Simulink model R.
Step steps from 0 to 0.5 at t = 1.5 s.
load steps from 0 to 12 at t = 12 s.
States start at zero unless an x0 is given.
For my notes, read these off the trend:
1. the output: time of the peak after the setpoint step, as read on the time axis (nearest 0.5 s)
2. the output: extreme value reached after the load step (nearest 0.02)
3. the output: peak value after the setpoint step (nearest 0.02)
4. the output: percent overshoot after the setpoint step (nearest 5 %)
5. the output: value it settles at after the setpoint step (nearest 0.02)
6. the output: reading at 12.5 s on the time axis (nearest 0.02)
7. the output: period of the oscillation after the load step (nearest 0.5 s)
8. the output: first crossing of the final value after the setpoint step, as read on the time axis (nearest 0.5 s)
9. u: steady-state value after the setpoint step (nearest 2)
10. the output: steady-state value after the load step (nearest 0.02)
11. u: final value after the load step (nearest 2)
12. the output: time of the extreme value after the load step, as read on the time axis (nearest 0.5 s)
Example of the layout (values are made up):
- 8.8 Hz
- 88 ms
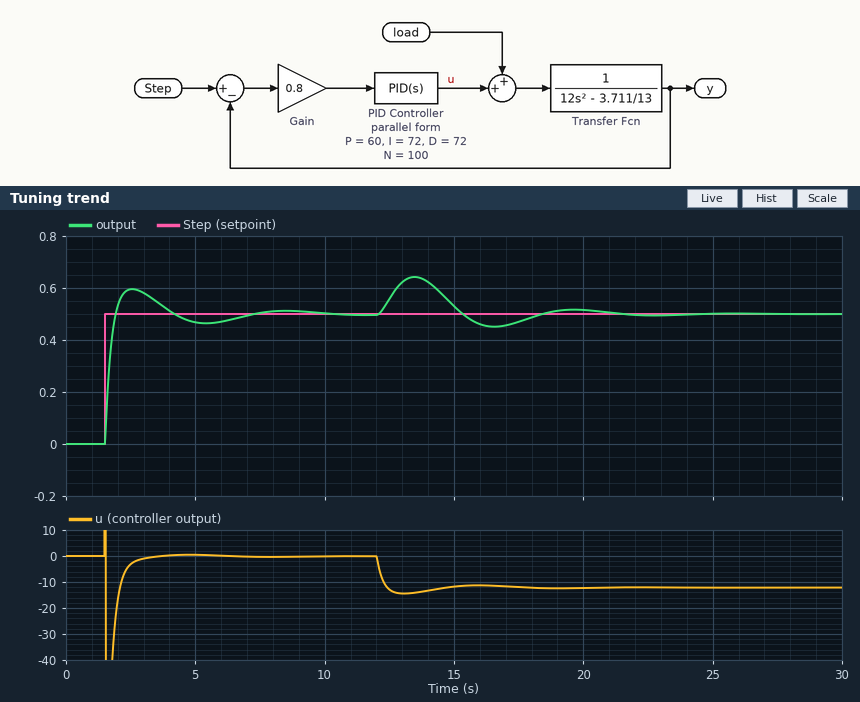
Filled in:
- 2.5 s
- 0.64
- 0.60
- 20 %
- 0.50
- 0.56
- 6.0 s
- 2.0 s
- 0
- 0.50
- -12
- 13.5 s
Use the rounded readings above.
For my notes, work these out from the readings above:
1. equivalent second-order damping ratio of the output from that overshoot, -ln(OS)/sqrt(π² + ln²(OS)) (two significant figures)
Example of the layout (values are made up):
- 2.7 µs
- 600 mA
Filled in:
- 0.46
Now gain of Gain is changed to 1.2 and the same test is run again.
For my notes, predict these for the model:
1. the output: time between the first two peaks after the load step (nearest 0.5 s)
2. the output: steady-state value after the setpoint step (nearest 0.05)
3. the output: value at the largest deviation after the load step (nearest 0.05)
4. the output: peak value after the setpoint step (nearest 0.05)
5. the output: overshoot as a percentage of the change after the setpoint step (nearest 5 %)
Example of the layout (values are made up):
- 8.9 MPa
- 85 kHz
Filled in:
- 6.5 s
- 0.50
- 0.60
- 0.55
- 15 %
